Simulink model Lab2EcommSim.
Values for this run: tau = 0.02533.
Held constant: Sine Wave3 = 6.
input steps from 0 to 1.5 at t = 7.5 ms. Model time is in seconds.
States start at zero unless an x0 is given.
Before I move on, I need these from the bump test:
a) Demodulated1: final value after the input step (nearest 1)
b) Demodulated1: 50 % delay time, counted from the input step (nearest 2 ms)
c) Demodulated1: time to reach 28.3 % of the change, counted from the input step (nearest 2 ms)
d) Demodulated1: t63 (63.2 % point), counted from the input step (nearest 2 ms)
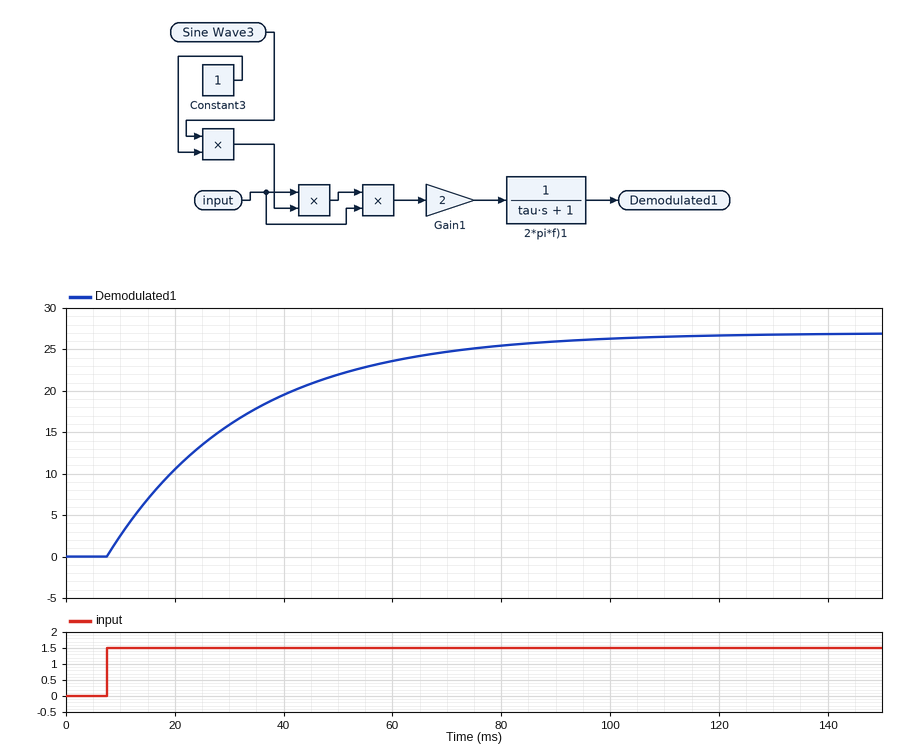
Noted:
27
18 ms
8 ms
26 ms
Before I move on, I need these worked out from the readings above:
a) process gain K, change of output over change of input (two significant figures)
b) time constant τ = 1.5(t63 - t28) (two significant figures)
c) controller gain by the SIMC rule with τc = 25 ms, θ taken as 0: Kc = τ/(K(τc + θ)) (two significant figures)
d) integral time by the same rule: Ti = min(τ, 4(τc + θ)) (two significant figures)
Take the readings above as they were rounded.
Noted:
18
27 ms
0.060
27 ms
